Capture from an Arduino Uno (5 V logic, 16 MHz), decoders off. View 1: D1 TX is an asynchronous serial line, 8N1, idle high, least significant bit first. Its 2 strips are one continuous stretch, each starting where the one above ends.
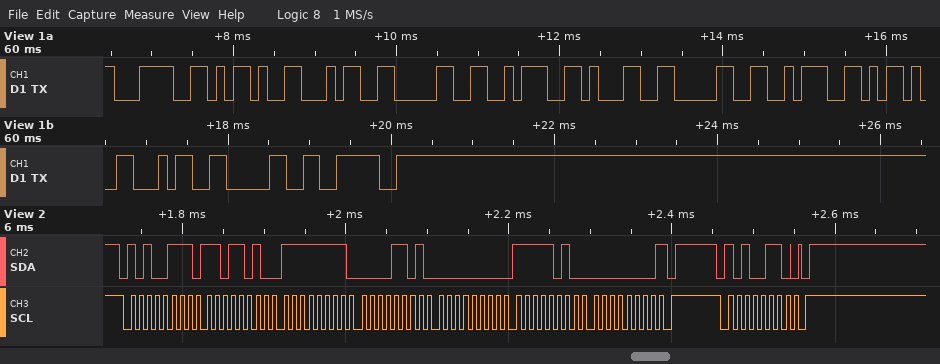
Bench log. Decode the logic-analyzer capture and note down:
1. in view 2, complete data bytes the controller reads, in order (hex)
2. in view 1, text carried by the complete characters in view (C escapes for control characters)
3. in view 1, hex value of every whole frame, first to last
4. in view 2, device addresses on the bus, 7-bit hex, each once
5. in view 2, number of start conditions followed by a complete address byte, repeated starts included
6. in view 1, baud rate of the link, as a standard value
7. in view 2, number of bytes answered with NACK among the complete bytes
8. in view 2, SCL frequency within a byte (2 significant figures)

DA FF 0D 00 FA 00
"<-40:10:-40>"
3C 2D 34 30 3A 31 30 3A 2D 34 30 3E
0x53
2
9600 baud
1
100 kHz
